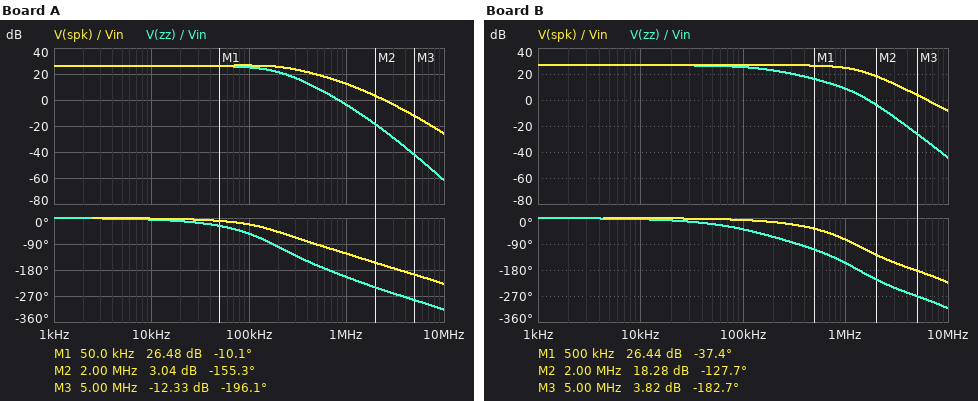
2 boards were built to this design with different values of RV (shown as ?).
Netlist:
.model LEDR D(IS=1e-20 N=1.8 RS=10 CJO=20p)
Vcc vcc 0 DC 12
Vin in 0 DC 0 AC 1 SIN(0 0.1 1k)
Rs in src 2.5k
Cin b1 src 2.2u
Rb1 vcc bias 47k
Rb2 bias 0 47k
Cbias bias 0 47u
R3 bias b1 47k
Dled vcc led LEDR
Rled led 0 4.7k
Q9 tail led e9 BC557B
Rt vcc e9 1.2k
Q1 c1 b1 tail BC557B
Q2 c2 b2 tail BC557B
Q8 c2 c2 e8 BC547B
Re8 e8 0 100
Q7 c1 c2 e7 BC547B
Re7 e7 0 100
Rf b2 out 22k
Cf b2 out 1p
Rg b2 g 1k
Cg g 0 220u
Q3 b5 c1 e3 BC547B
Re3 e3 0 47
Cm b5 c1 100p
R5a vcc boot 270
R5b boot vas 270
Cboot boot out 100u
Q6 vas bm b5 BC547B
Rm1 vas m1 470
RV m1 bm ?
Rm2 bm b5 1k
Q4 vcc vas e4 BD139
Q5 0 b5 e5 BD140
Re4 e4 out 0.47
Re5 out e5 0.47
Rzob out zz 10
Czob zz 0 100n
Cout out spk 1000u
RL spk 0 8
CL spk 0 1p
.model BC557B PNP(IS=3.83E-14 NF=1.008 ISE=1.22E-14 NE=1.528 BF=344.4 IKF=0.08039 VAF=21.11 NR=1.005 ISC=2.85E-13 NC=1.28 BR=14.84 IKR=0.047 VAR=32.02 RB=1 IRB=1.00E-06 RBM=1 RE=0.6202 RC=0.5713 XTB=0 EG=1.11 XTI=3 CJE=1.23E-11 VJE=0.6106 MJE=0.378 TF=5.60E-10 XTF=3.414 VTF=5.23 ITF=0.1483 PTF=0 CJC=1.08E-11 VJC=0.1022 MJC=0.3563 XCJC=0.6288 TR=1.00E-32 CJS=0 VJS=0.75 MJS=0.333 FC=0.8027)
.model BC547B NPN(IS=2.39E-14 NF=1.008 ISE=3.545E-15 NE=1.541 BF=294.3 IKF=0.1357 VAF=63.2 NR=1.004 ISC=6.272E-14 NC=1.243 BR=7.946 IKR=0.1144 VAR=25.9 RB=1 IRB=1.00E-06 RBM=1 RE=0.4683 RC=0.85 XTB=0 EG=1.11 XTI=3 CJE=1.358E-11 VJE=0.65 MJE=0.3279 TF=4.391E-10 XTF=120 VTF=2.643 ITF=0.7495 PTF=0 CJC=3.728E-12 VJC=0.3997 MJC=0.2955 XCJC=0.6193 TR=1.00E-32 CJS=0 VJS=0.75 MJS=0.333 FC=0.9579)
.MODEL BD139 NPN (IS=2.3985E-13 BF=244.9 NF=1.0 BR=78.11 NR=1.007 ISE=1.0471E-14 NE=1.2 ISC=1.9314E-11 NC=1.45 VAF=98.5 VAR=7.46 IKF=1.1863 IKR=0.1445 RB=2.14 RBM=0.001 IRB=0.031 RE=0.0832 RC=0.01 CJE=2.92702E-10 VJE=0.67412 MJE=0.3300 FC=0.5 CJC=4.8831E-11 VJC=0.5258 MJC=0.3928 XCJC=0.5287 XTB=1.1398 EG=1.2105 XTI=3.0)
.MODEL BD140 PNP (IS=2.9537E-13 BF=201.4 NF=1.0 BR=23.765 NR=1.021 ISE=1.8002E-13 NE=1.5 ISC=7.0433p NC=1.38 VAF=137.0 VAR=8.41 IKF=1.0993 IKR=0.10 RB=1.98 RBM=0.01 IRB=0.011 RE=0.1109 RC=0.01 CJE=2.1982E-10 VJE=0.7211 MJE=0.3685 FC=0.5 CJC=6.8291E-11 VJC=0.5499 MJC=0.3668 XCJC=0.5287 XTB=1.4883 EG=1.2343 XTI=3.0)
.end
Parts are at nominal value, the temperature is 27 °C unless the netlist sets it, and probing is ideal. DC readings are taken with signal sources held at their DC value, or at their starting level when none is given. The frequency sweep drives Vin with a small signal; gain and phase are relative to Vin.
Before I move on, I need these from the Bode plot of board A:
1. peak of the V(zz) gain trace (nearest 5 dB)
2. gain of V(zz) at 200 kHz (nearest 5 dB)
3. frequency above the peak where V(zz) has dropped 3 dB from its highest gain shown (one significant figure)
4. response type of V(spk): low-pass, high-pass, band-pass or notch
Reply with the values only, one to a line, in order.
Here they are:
25 dB
20 dB
200 kHz
low-pass
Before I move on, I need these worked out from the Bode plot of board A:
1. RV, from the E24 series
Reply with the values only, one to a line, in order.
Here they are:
120 Ω
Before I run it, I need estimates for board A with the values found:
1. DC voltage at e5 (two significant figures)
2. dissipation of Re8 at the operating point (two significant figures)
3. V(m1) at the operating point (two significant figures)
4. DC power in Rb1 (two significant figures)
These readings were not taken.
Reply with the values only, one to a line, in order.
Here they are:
6.1 V
25 µW
6.3 V
760 µW
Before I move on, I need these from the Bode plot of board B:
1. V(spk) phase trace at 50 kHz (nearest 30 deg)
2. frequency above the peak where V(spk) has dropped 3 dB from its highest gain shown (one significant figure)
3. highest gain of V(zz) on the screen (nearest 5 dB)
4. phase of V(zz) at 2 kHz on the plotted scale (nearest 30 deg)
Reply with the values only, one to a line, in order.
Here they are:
0 deg
1 MHz
25 dB
0 deg
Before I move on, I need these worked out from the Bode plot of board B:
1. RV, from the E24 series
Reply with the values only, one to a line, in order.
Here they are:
430 Ω
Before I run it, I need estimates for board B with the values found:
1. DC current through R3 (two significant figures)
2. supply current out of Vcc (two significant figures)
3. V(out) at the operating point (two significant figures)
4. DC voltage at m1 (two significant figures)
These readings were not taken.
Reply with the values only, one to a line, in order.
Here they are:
1.3 µA
45 mA
6.1 V
6.4 V
